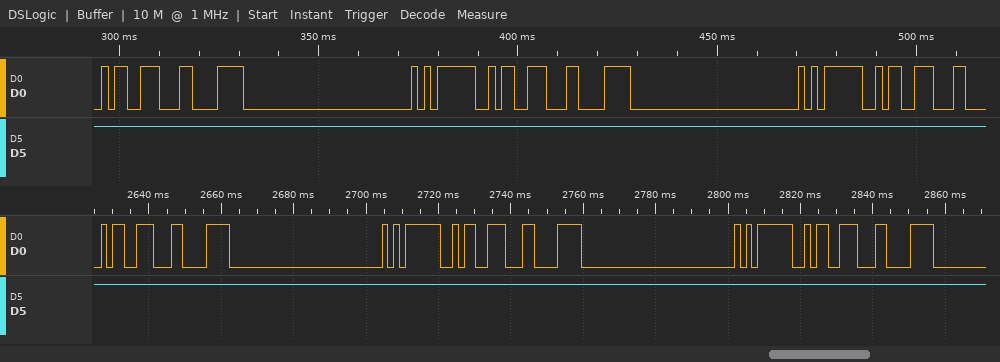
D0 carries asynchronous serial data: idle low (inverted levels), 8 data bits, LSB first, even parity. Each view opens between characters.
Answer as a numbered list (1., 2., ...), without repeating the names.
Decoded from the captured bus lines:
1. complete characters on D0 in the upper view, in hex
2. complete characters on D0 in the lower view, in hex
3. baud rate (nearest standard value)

1. 19, 1E, 05, 19, 1E, 05, 19
2. 19, 1E, 05, 19, 1E, 05, 19, 1E
3. 600 baud
